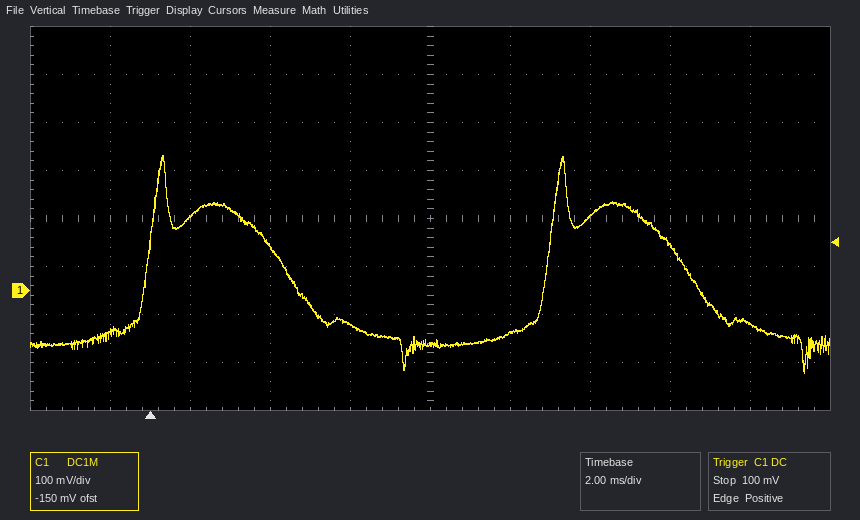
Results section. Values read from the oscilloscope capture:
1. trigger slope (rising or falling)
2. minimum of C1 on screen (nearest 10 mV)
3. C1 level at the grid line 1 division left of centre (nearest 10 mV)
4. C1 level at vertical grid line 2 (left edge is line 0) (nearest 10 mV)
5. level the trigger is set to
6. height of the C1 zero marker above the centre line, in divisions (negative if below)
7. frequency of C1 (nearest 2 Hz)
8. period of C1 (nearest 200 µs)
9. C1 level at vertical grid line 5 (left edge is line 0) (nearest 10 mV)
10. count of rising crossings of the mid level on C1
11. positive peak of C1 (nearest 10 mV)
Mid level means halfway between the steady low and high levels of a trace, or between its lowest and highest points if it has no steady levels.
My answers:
rising
-170 mV
-70 mV
150 mV
100 mV
-1.5 div
100 Hz
10.0 ms
-110 mV
2
280 mV
